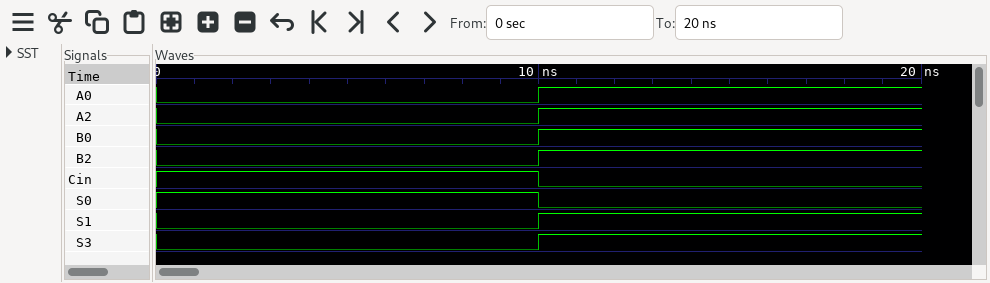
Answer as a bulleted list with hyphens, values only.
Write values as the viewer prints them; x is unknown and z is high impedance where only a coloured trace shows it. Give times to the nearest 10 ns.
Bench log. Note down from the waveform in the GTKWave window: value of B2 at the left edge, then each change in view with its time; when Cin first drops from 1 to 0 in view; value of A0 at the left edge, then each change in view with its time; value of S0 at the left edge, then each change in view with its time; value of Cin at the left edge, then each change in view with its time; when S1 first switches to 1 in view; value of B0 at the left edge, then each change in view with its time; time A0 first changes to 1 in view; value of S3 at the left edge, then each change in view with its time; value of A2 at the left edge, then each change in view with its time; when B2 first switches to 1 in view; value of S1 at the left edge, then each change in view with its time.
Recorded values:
- 0, 1 at 10 ns
- 10 ns
- 0, 1 at 10 ns
- 1, 0 at 10 ns
- 1, 0 at 10 ns
- 10 ns
- 0, 1 at 10 ns
- 10 ns
- 0, 1 at 10 ns
- 0, 1 at 10 ns
- 10 ns
- 0, 1 at 10 ns
